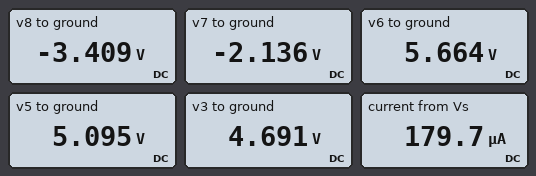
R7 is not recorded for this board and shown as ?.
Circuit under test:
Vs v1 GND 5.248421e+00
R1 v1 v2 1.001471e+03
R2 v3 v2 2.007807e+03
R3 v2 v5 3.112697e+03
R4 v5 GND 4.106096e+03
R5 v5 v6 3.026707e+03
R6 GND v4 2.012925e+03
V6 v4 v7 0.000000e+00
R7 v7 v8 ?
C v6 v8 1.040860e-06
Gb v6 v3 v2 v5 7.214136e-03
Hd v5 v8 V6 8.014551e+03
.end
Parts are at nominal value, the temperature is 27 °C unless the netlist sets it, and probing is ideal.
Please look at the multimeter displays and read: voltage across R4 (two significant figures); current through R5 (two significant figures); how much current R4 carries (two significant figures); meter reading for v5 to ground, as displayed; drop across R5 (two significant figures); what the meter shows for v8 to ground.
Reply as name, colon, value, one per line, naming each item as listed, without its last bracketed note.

voltage across R4: 5.1 V
current through R5: 190 µA
how much current R4 carries: 1.2 mA
meter reading for v5 to ground, as displayed: 5.095 V
drop across R5: 570 mV
what the meter shows for v8 to ground: -3.409 V
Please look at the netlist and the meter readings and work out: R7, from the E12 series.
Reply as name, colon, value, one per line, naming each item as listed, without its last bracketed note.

R7, from the E12 series: 1.2 kΩ
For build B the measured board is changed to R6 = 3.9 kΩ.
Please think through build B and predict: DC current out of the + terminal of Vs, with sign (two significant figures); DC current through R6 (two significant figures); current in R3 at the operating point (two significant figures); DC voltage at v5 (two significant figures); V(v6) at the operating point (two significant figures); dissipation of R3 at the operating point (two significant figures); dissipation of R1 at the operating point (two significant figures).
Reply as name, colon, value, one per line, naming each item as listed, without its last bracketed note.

DC current out of the + terminal of Vs, with sign: -570 µA
DC current through R6: 2.0 mA
current in R3 at the operating point: 27 µA
DC voltage at v5: 5.7 V
V(v6) at the operating point: 3.9 V
dissipation of R3 at the operating point: 2.2 µW
dissipation of R1 at the operating point: 330 µW
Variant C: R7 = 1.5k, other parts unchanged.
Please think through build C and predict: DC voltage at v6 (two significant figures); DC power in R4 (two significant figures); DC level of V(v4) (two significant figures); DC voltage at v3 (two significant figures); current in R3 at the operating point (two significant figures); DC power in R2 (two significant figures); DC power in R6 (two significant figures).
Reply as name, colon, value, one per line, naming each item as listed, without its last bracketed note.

DC voltage at v6: 5.5 V
DC power in R4: 6.5 mW
DC level of V(v4): -2.3 V
DC voltage at v3: 4.9 V
current in R3 at the operating point: 5.1 µA
DC power in R2: 27 µW
DC power in R6: 2.6 mW
